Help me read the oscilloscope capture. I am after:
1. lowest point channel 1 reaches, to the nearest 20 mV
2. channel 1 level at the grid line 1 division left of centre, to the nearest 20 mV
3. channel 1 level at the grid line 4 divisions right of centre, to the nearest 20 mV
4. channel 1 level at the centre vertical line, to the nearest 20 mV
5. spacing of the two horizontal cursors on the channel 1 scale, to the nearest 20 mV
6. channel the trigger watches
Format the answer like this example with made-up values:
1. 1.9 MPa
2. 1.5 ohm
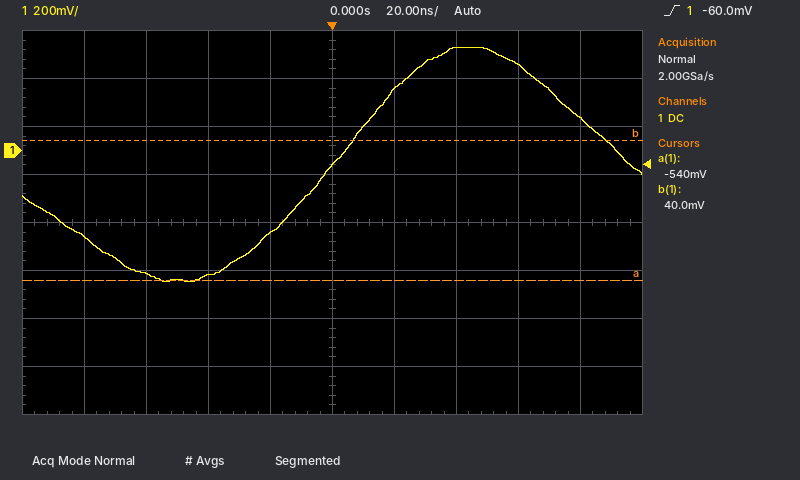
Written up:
1. -540 mV
2. -340 mV
3. 140 mV
4. -60 mV
5. 580 mV
6. channel 1
